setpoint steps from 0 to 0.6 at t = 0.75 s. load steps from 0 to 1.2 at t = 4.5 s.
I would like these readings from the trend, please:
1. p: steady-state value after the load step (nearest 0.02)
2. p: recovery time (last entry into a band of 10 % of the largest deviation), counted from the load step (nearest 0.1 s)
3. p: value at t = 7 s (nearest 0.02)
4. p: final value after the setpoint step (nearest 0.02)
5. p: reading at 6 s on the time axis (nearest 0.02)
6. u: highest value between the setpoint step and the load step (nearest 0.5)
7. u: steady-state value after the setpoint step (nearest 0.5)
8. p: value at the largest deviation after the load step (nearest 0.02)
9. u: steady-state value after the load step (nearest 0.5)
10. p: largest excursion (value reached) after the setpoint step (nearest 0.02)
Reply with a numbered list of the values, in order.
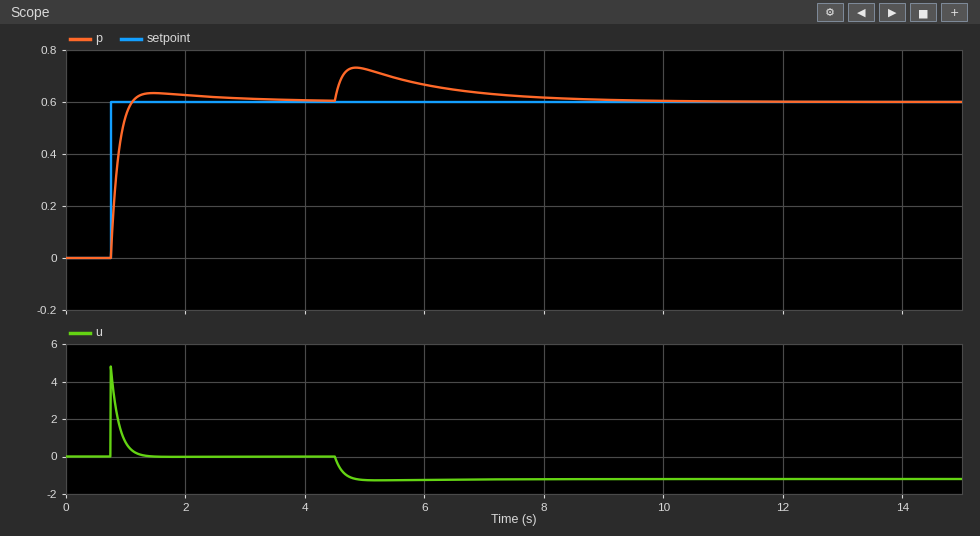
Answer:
1. 0.60
2. 3.9 s
3. 0.64
4. 0.60
5. 0.66
6. 5.0
7. 0.0
8. 0.74
9. -1.0
10. 0.64
